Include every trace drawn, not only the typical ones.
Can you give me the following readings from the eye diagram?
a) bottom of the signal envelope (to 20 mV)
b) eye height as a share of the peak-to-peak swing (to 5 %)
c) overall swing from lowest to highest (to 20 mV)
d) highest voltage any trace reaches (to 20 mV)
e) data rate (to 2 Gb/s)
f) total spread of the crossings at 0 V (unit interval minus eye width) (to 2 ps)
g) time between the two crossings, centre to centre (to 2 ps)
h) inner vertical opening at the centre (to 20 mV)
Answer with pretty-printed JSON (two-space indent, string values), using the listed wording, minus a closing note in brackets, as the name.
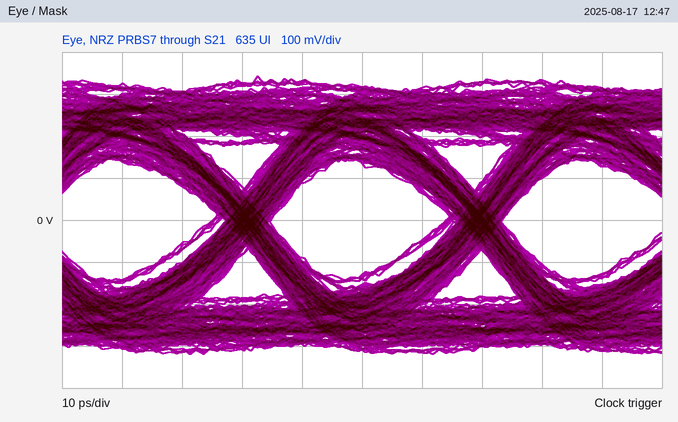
{
  "bottom of the signal envelope": "-320 mV",
  "eye height as a share of the peak-to-peak swing": "40 %",
  "overall swing from lowest to highest": "660 mV",
  "highest voltage any trace reaches": "340 mV",
  "data rate": "26 Gb/s",
  "total spread of the crossings at 0 V (unit interval minus eye width)": "10 ps",
  "time between the two crossings, centre to centre": "38 ps",
  "inner vertical opening at the centre": "260 mV"
}
